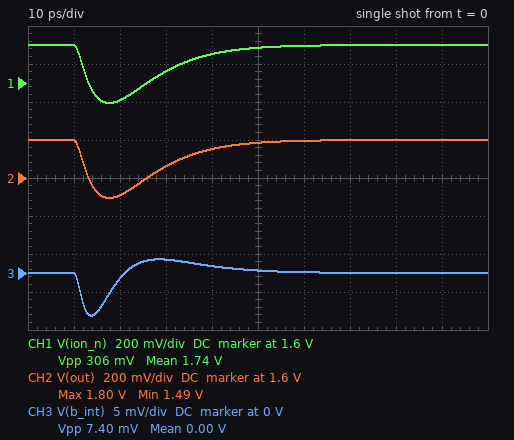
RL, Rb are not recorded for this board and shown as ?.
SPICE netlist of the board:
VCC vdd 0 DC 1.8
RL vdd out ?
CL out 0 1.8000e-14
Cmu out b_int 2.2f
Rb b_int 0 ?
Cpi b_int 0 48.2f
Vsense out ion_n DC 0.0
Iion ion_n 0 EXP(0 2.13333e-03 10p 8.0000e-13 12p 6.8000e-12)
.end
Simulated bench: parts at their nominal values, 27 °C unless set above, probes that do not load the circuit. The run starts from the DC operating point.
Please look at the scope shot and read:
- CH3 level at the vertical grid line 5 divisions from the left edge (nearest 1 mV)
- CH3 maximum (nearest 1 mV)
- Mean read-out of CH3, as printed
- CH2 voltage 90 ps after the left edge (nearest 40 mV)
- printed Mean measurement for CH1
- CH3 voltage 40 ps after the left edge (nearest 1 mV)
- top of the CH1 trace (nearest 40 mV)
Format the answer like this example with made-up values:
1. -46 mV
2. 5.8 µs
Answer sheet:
1. 0 V
2. 2 mV
3. 0.00 V
4. 1.80 V
5. 1.74 V
6. 1 mV
7. 1.80 V
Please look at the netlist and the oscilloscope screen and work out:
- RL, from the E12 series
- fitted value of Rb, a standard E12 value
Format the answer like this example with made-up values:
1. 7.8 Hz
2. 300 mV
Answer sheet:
1. 330 Ω
2. 56 Ω
